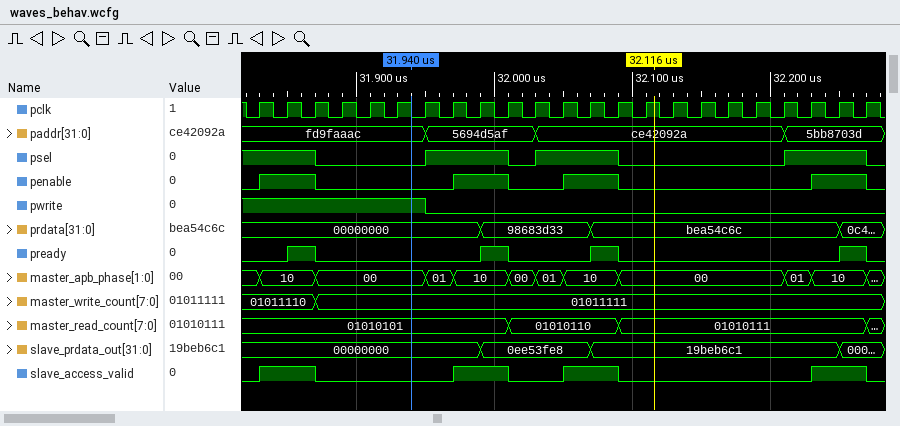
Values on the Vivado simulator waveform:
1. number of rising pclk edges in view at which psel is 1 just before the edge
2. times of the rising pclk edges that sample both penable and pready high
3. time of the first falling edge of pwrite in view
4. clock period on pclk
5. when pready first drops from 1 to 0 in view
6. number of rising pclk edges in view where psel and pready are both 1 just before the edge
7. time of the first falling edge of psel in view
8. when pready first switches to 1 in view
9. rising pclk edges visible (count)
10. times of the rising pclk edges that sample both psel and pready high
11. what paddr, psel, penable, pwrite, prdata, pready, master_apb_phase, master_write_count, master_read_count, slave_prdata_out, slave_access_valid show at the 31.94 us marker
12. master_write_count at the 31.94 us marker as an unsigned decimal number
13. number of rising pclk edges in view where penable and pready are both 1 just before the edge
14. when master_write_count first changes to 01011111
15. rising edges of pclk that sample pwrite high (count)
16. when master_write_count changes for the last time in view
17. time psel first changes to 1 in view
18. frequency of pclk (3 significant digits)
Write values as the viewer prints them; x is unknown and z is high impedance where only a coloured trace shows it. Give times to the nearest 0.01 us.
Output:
12
31.87 us, 32.01 us, 32.09 us, 32.27 us
31.95 us
0.02 us
31.87 us
4
31.87 us
31.85 us
23
31.87 us, 32.01 us, 32.09 us, 32.27 us
paddr=fd9faaac, psel=0, penable=0, pwrite=1, prdata=00000000, pready=0, master_apb_phase=00, master_write_count=01011111, master_read_count=01010101, slave_prdata_out=00000000, slave_access_valid=0
95
4
31.87 us
7
31.87 us
31.95 us
50.0 MHz
